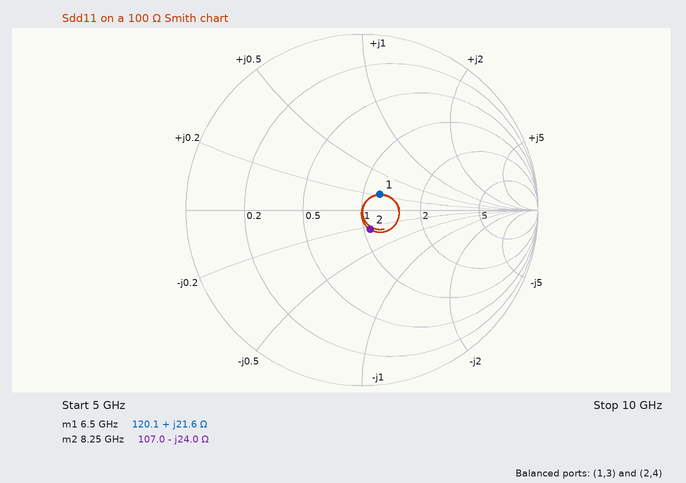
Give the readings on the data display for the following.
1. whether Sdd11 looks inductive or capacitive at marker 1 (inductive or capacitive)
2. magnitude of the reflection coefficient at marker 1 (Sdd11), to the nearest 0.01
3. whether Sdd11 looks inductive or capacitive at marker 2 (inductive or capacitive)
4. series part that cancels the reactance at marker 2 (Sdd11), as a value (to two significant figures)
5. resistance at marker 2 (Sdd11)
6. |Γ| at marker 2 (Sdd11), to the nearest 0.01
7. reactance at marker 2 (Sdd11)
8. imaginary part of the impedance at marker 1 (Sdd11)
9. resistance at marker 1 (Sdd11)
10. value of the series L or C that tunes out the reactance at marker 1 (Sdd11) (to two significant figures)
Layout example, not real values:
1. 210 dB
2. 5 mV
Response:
1. inductive
2. 0.13
3. capacitive
4. 460 pH
5. 107.0 Ω
6. 0.12
7. -24.0 Ω
8. +21.6 Ω
9. 120.1 Ω
10. 1.1 pF
